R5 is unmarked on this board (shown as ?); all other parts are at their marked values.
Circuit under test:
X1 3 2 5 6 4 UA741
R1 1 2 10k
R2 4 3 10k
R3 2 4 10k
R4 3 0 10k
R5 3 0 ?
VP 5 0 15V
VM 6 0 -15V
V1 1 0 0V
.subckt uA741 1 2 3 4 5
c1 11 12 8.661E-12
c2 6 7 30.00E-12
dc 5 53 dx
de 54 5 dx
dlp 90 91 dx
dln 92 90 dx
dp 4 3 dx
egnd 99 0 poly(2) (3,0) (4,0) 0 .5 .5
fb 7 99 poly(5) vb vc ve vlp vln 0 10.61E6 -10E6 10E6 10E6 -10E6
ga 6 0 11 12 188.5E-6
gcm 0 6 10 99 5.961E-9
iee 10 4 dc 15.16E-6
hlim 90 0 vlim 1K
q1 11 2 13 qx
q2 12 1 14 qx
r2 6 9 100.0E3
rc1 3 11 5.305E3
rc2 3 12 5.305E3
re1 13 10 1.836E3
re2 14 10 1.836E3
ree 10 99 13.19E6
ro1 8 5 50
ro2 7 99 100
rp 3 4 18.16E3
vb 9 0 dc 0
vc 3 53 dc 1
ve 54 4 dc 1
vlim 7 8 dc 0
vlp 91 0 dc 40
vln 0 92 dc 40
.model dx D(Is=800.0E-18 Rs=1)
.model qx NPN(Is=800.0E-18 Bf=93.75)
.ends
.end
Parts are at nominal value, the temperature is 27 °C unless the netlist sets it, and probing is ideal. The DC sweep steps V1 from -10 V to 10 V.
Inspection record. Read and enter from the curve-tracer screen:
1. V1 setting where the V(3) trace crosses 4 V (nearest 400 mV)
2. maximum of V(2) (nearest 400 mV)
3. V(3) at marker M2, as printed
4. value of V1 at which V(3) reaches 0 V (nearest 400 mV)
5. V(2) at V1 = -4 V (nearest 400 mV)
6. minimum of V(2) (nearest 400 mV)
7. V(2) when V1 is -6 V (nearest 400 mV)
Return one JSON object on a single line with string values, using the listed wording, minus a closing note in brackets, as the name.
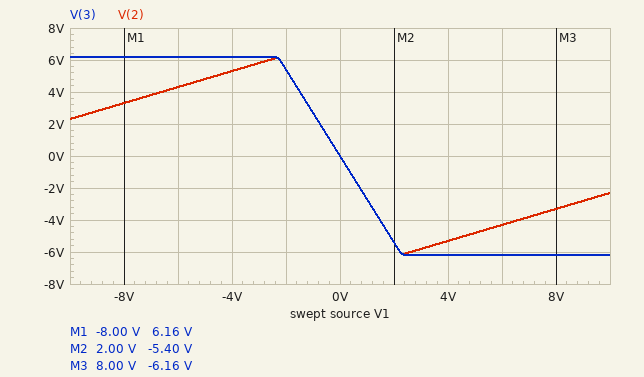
{"V1 setting where the V(3) trace crosses 4 V": "-1.6 V", "maximum of V(2)": "6.0 V", "V(3) at marker M2, as printed": "-5.40 V", "value of V1 at which V(3) reaches 0 V": "0 V", "V(2) at V1 = -4 V": "5.2 V", "minimum of V(2)": "-6.0 V", "V(2) when V1 is -6 V": "4.4 V"}
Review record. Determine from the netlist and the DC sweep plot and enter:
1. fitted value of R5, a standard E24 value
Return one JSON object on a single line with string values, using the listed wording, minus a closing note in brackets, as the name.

{"fitted value of R5, a standard E24 value": "27 kΩ"}
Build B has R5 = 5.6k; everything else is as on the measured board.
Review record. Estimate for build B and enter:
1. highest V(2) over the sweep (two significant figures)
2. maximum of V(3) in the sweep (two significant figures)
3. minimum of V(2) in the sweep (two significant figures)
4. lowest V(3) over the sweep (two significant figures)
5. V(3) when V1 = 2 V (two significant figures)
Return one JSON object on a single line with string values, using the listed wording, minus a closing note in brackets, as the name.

{"highest V(2) over the sweep": "3.8 V", "maximum of V(3) in the sweep": "3.9 V", "minimum of V(2) in the sweep": "-3.8 V", "lowest V(3) over the sweep": "-3.9 V", "V(3) when V1 = 2 V": "-1.1 V"}
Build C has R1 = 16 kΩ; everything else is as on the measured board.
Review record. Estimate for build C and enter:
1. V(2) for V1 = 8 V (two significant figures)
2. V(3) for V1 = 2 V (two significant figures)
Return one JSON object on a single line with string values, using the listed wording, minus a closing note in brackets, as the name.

{"V(2) for V1 = 8 V": "-5.9 V", "V(3) for V1 = 2 V": "-1.7 V"}
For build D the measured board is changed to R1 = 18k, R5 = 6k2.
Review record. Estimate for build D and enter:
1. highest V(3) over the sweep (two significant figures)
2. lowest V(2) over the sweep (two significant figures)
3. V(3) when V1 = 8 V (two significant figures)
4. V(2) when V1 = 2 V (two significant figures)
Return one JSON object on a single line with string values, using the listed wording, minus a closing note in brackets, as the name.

{"highest V(3) over the sweep": "2.7 V", "lowest V(2) over the sweep": "-2.7 V", "V(3) when V1 = 8 V": "-2.2 V", "V(2) when V1 = 2 V": "-540 mV"}
